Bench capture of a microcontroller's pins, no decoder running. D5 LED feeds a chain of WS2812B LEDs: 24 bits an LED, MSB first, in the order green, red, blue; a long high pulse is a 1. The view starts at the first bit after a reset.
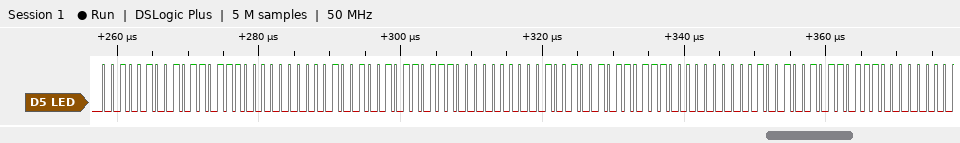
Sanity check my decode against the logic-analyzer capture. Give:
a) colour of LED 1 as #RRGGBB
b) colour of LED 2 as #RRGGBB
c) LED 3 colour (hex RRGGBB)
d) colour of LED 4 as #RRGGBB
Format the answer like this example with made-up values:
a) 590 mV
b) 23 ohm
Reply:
a) #B72400
b) #B72400
c) #B72400
d) #B72400
